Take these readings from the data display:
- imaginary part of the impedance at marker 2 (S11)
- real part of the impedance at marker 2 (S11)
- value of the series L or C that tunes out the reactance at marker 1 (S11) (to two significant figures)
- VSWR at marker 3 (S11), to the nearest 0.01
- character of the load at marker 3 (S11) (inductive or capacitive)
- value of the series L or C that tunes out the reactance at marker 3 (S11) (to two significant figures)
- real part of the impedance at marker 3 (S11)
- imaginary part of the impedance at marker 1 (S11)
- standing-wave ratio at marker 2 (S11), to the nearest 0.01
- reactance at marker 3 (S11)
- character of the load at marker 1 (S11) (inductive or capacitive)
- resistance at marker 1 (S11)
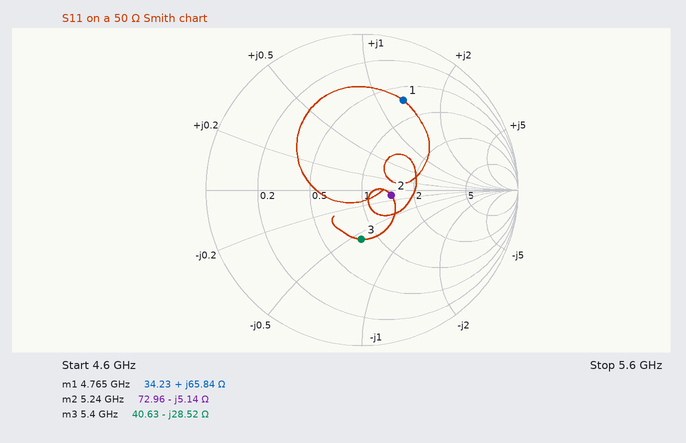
-5.14 Ω
72.96 Ω
510 fF
1.92
capacitive
840 pH
40.63 Ω
+65.84 Ω
1.47
-28.52 Ω
inductive
34.23 Ω
